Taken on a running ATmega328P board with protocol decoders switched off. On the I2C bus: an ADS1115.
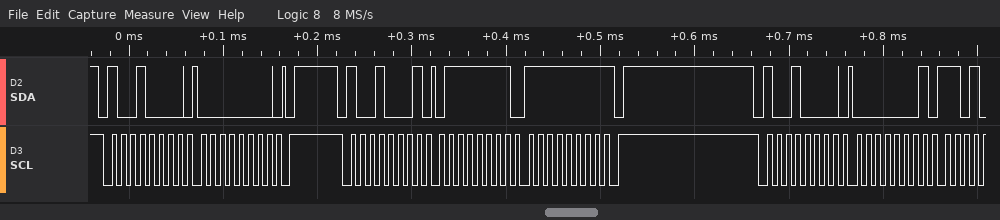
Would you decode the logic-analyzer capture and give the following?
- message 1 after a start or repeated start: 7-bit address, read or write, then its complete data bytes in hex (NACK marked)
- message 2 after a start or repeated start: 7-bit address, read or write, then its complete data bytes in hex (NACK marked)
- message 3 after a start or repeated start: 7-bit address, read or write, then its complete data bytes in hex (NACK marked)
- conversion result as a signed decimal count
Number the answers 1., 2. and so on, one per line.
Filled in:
1. 0x48 write: 00
2. 0x48 read: 7F FF NACK
3. 0x48 write: 01
4. 32767
